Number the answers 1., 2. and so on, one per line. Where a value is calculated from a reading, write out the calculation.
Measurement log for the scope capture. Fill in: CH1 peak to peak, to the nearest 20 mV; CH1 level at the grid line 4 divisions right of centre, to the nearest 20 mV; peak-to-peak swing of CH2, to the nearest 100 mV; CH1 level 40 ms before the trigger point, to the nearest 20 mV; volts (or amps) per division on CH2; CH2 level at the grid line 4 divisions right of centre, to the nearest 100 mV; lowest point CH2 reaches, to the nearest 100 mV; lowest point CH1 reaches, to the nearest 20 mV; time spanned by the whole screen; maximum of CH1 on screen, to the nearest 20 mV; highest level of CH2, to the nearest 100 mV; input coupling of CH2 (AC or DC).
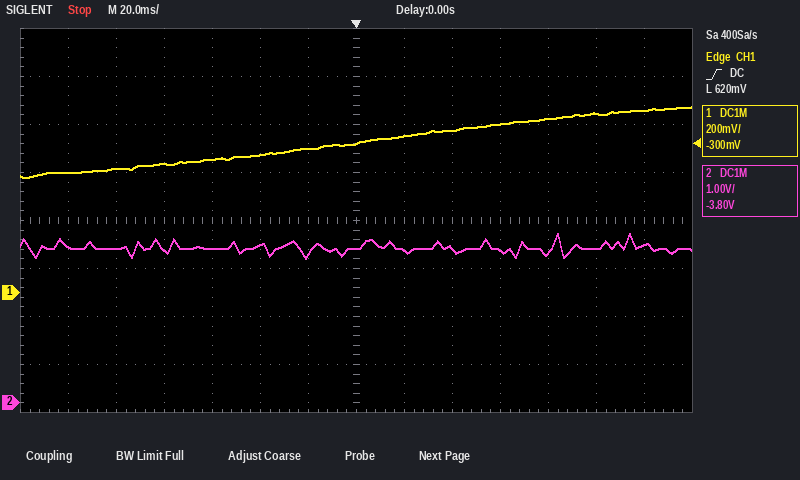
1. 780 mV − (480 mV) = 300 mV
2. 720 mV
3. 3.5 V − (3.0 V) = 500 mV
4. 580 mV
5. 1 V
6. 3.1 V
7. 3.0 V
8. 480 mV
9. 280 ms
10. 780 mV
11. 3.5 V
12. DC
